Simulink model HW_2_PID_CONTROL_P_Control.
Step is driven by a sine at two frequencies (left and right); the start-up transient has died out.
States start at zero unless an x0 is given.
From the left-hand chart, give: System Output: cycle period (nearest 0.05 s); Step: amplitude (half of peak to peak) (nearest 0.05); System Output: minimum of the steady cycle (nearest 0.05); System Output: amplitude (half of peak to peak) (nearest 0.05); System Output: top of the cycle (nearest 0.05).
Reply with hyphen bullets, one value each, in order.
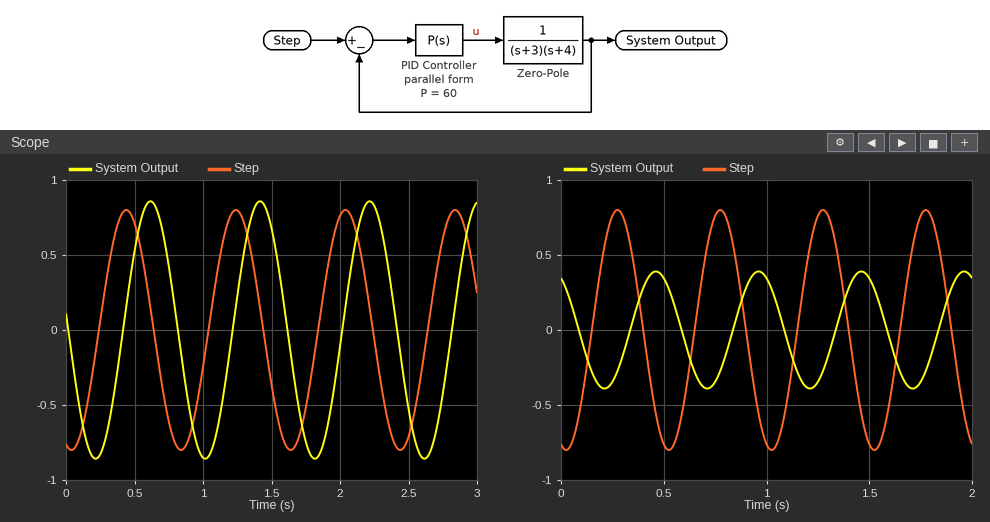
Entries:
- 0.80 s
- 0.80
- -0.85
- 0.85
- 0.85
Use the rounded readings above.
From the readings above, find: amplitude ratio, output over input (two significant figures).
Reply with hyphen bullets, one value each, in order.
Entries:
- 1.1
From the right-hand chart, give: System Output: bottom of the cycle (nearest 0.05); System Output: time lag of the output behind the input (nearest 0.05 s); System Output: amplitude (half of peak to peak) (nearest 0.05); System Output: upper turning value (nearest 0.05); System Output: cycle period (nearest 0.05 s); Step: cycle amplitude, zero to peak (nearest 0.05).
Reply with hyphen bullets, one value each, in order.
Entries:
- -0.40
- 0.20 s
- 0.40
- 0.40
- 0.50 s
- 0.80
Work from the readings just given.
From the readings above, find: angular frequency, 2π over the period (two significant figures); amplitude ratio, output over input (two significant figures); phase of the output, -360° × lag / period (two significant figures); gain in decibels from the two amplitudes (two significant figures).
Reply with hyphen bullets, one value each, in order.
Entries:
- 13 rad/s
- 0.50
- -140°
- -6.0 dB
